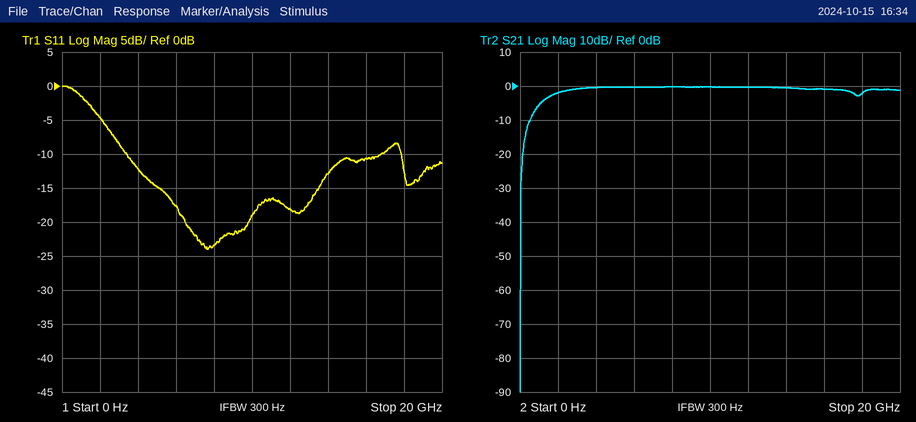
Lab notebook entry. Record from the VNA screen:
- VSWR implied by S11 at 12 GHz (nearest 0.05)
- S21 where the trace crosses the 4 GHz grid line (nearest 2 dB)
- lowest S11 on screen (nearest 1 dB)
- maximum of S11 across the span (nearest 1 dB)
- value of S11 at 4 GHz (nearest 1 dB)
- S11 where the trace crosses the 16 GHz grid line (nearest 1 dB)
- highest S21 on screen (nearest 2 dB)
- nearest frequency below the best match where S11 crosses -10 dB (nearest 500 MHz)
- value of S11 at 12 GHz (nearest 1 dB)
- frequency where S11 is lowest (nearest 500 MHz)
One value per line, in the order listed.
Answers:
1.30
0 dB
-24 dB
0 dB
-12 dB
-11 dB
0 dB
3.5 GHz
-18 dB
7.5 GHz
